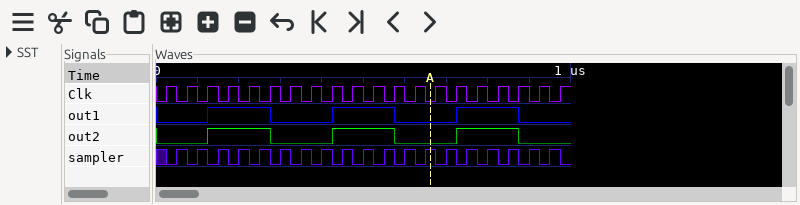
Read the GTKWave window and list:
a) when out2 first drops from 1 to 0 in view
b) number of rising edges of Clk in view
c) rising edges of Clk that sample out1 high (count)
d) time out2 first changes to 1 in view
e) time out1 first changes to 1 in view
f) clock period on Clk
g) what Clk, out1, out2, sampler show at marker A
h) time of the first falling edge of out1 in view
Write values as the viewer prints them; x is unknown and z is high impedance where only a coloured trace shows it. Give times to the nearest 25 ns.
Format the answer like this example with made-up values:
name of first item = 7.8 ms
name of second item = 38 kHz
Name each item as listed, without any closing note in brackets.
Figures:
when out2 first drops from 1 to 0 in view = 275 ns
number of rising edges of Clk in view = 20
rising edges of Clk that sample out1 high = 9
time out2 first changes to 1 in view = 125 ns
time out1 first changes to 1 in view = 125 ns
clock period on Clk = 50 ns
what Clk, out1, out2, sampler show at marker A = Clk=0, out1=0, out2=0, sampler=1
time of the first falling edge of out1 in view = 275 ns
